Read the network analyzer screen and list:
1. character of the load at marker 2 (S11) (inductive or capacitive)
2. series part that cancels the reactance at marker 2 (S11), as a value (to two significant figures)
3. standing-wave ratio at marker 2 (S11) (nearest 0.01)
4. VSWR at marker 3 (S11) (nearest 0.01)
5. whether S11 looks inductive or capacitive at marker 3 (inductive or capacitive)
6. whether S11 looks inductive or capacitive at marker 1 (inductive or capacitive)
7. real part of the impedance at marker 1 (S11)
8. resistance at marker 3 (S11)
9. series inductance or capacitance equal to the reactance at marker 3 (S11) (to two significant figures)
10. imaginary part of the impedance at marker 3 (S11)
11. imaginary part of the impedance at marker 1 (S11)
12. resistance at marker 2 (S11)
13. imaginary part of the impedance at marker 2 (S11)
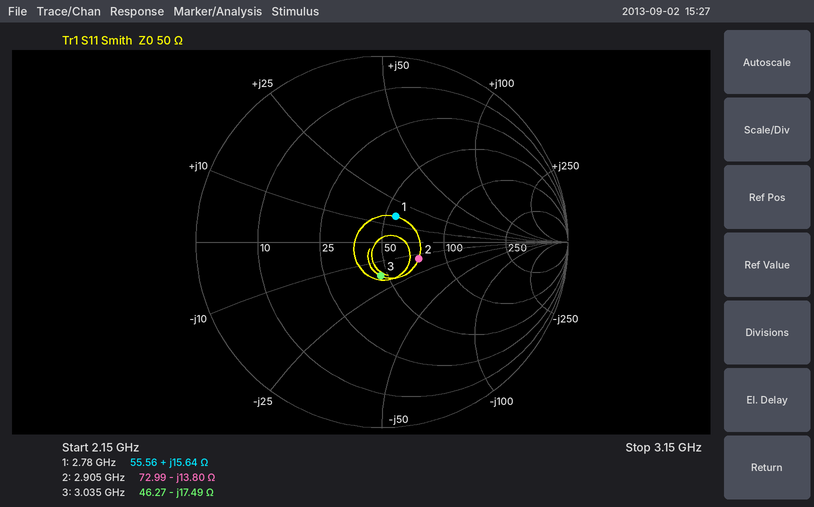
capacitive
760 pH
1.55
1.45
capacitive
inductive
55.56 Ω
46.27 Ω
3.0 pF
-17.49 Ω
+15.64 Ω
72.99 Ω
-13.80 Ω
